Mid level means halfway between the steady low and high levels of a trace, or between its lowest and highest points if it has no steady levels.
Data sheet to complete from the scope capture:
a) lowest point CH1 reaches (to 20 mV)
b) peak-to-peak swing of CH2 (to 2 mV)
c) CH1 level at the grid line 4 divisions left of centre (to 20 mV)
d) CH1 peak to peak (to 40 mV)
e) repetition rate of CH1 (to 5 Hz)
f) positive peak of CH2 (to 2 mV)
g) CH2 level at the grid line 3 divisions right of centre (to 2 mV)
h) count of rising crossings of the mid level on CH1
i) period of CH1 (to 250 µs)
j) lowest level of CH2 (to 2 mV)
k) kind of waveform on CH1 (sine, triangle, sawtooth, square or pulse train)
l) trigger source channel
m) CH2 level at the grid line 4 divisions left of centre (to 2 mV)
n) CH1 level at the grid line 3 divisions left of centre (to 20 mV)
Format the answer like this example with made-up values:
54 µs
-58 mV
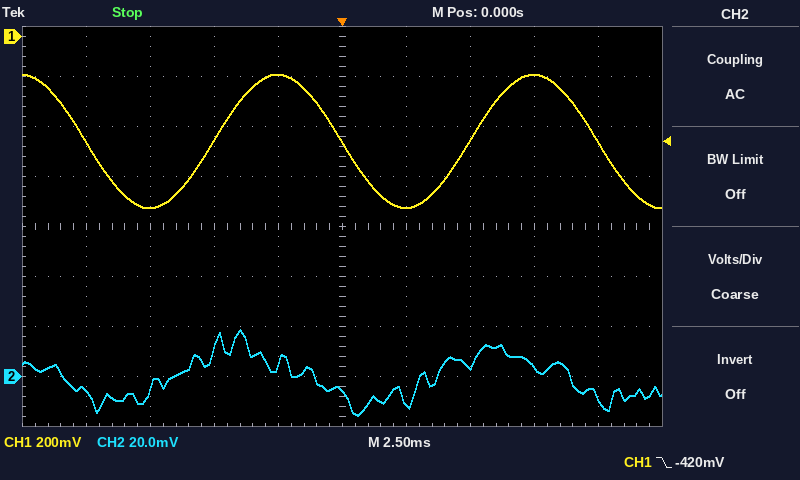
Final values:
-680 mV
34 mV
-420 mV
520 mV
100 Hz
18 mV
4 mV
2
10.00 ms
-16 mV
sine
CH1
-6 mV
-680 mV
